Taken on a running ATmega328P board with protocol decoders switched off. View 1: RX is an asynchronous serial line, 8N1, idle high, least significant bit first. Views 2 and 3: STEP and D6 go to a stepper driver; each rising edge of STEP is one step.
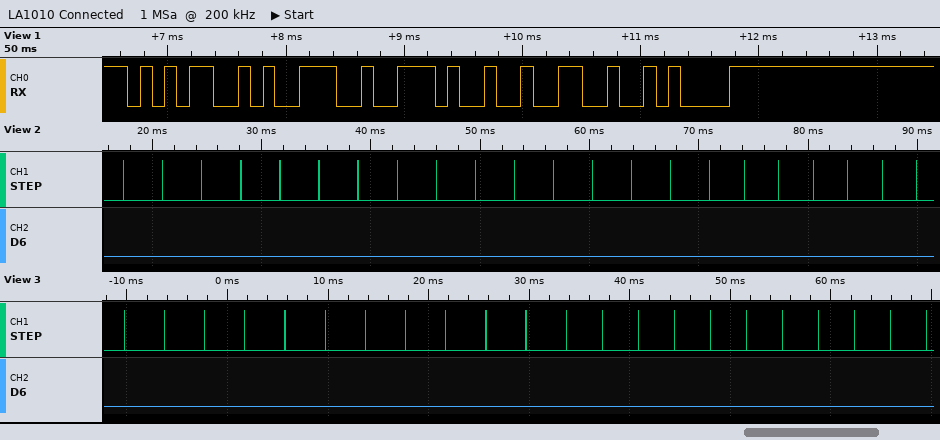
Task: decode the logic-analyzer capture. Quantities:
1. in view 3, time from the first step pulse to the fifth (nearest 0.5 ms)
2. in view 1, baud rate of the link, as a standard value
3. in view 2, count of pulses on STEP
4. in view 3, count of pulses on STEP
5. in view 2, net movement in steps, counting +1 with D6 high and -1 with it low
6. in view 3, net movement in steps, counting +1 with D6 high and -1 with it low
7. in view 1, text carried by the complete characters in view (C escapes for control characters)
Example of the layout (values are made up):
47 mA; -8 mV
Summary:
16.0 ms; 9600 baud; 22; 22; -22; -22; "59.2\n"
